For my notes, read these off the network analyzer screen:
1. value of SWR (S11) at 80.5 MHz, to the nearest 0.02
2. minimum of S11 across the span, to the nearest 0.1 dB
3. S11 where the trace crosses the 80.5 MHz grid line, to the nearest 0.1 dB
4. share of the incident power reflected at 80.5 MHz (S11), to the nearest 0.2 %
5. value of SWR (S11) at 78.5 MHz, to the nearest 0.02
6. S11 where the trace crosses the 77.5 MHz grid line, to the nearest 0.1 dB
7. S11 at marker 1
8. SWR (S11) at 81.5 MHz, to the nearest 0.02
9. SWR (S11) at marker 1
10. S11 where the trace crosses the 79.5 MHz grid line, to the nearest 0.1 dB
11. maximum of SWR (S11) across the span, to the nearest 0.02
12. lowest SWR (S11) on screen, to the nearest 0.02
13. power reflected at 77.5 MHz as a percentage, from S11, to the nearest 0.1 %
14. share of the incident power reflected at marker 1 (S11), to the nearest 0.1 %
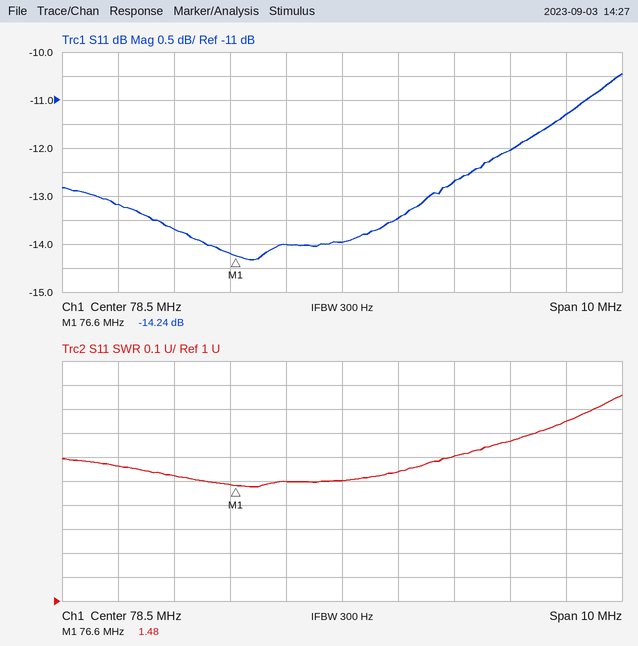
1.60
-14.3 dB
-12.7 dB
5.4 %
1.50
-14.0 dB
-14.24 dB
1.66
1.48
-13.5 dB
1.86
1.48
4.0 %
3.8 %
